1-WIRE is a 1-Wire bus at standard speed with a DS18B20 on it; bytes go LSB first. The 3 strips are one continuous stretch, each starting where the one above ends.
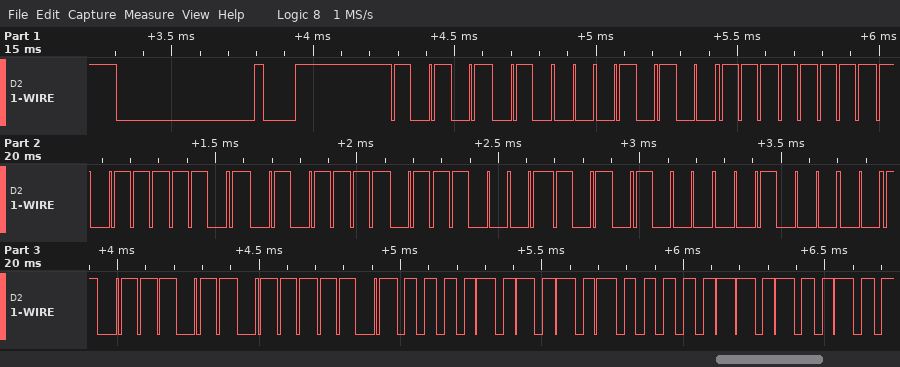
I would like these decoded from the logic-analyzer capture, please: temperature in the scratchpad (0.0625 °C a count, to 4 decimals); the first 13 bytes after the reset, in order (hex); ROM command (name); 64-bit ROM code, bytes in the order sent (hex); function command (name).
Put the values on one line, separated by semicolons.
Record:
85.0000 °C; 55 28 FF 7D F5 8E 15 04 DD BE 50 05 4B; Match ROM; 28 FF 7D F5 8E 15 04 DD; Read Scratchpad
